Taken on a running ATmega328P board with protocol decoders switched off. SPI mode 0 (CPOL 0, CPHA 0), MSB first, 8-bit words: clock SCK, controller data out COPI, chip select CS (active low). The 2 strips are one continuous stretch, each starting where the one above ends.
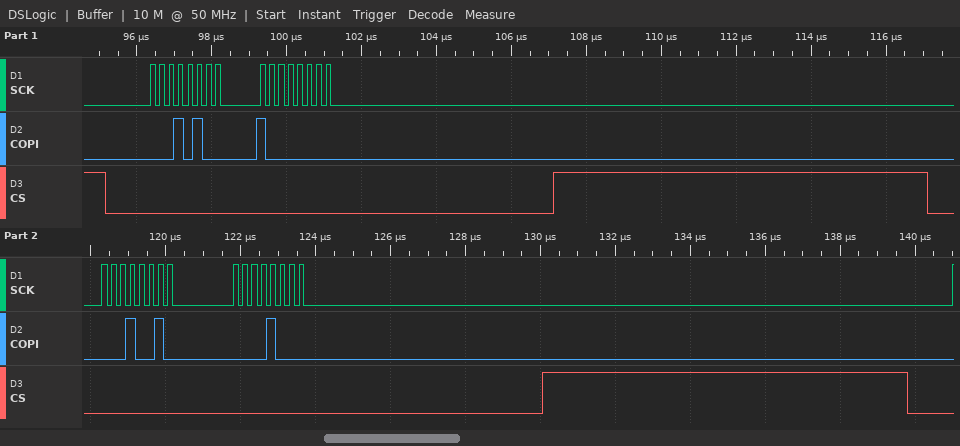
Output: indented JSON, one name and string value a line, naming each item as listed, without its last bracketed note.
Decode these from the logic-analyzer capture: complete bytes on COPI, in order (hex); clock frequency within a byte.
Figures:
{
  "complete bytes on COPI, in order": "14 80 12 08",
  "clock frequency within a byte": "4 MHz"
}
